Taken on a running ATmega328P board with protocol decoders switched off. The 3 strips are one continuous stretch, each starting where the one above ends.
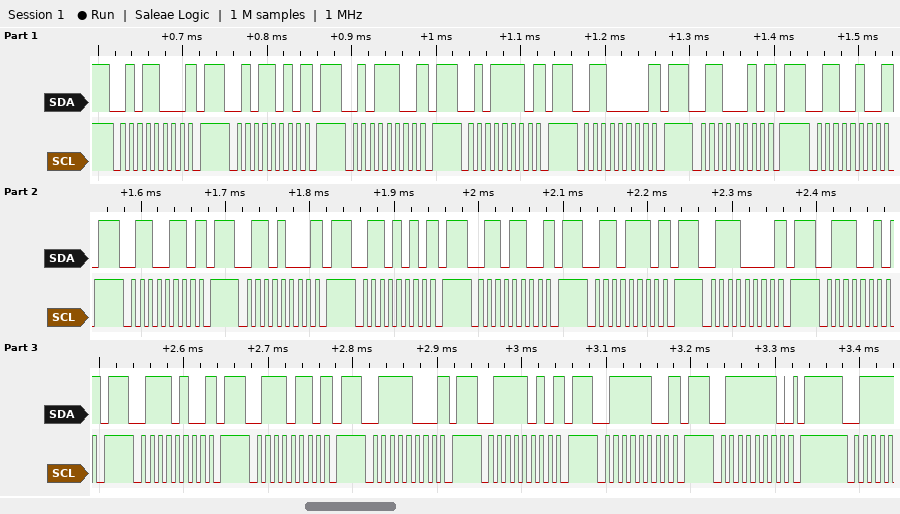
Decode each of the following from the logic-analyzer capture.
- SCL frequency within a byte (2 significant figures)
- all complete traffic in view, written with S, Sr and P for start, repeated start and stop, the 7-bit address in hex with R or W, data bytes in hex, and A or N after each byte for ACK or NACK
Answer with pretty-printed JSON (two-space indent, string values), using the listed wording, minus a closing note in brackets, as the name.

{
  "SCL frequency within a byte": "100 kHz",
  "all complete traffic in view, written with S, Sr and P for start, repeated start and stop, the 7-bit address in hex with R or W, data bytes in hex, and A or N after each byte for ACK or NACK": "S 2CW N P S 2DW N P S 2EW N P S 2FW N P S 30W N P S 31W N P S 32W N P S 33W N P S 34W N P S 35W N P S 36W N P S 37W N P S 38W N P S 39W N P S 3AW N P S 3BW N P S 3CW N P S 3DW N P S 3EW N P S 3FW A P"
}
